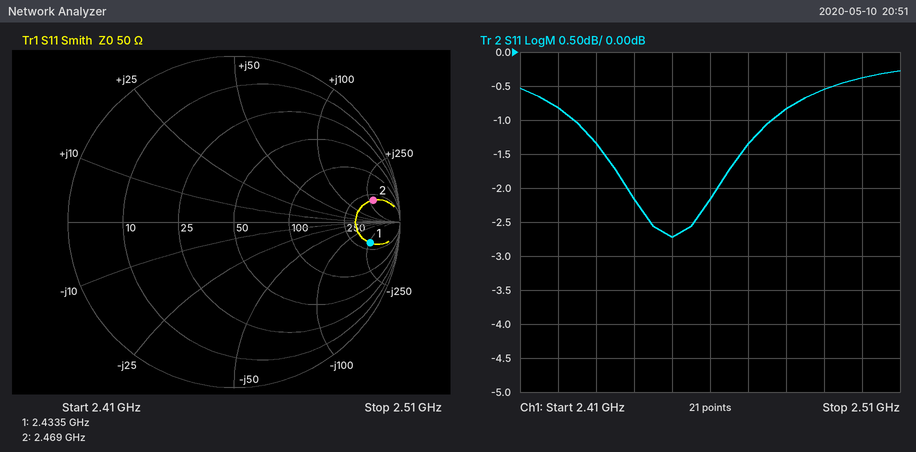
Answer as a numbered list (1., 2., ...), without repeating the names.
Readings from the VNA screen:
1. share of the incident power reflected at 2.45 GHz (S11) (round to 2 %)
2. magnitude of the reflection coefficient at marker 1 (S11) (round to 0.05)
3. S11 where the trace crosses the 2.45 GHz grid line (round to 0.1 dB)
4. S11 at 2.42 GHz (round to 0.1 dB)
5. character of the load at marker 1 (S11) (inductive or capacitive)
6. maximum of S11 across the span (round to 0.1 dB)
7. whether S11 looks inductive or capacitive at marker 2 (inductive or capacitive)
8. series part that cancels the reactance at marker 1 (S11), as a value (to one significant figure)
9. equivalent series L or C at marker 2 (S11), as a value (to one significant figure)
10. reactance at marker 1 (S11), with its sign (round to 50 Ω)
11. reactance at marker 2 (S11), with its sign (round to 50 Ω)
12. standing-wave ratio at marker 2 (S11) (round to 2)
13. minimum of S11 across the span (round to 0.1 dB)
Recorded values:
1. 54 %
2. 0.85
3. -2.7 dB
4. -0.8 dB
5. capacitive
6. -0.3 dB
7. inductive
8. 20 nH
9. 20 nH
10. -250 Ω
11. +300 Ω
12. 12
13. -2.7 dB
